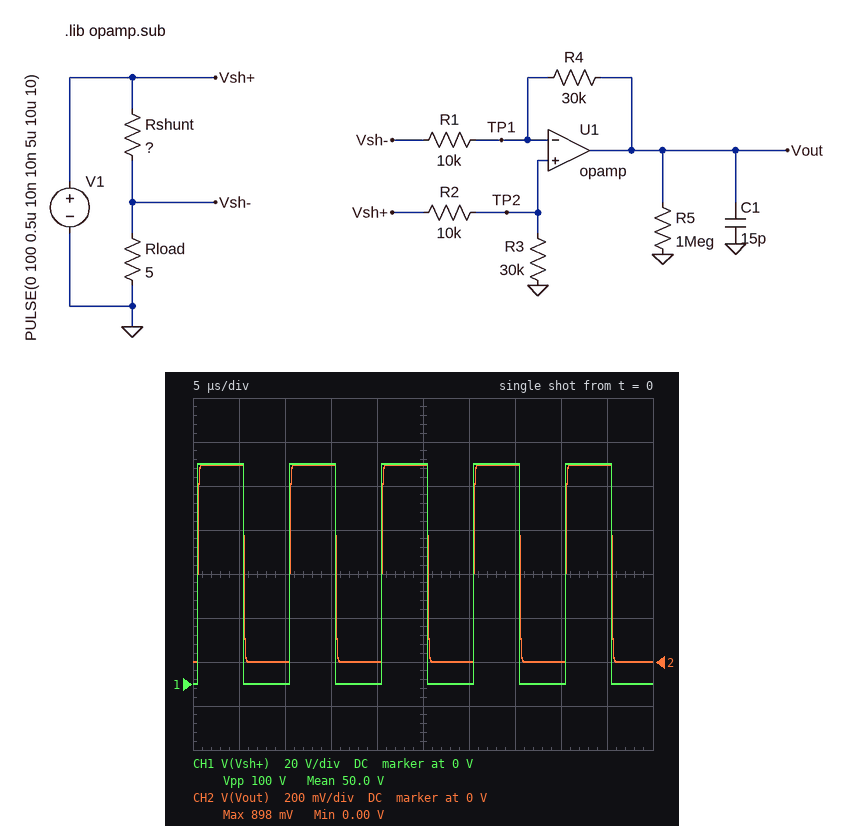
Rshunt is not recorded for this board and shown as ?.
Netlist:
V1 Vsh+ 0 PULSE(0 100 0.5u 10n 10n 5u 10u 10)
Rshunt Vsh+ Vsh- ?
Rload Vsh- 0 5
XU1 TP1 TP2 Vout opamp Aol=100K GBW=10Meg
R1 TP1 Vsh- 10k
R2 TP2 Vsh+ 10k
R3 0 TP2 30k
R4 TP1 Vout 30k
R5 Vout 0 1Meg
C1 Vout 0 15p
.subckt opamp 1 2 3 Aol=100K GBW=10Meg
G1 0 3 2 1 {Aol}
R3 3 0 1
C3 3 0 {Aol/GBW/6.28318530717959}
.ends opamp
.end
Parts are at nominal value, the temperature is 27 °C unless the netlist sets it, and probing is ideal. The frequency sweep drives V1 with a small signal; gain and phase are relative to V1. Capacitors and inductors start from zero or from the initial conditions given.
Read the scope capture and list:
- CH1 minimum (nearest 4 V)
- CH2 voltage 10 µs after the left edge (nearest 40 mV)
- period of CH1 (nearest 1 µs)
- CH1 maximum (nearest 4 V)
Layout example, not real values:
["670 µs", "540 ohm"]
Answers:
["0 V", "0 V", "10 µs", "100 V"]
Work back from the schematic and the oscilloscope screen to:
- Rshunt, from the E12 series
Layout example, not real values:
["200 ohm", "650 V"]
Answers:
["0.015 Ω"]
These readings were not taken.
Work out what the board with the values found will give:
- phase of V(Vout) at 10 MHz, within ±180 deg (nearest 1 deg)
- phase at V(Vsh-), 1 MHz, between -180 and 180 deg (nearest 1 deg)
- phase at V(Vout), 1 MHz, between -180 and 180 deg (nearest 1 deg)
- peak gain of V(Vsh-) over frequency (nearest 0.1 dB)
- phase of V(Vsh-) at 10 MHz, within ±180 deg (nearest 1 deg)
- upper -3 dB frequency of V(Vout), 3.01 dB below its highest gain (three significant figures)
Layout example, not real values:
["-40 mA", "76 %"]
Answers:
["-76 deg", "0 deg", "-22 deg", "0 dB", "0 deg", "2.50 MHz"]
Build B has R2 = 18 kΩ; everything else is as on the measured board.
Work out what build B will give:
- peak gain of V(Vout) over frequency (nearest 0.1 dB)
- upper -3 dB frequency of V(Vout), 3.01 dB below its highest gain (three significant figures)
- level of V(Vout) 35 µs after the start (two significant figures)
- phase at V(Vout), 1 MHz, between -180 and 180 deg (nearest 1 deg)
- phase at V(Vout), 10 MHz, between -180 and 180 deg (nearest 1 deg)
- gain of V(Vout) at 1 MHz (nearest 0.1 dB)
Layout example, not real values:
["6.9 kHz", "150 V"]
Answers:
["-6.2 dB", "2.50 MHz", "-49 V", "158 deg", "104 deg", "-6.8 dB"]
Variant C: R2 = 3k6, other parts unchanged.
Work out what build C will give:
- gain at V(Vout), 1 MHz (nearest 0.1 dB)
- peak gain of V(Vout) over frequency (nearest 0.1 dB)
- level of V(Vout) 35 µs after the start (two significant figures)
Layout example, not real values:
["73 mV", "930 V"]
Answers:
["-5.4 dB", "-4.7 dB", "58 V"]
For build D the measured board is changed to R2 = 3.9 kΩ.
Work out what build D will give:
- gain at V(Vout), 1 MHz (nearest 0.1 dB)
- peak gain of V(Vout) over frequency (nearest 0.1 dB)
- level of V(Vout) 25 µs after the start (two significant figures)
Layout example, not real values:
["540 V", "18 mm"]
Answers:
["-5.9 dB", "-5.2 dB", "55 V"]
